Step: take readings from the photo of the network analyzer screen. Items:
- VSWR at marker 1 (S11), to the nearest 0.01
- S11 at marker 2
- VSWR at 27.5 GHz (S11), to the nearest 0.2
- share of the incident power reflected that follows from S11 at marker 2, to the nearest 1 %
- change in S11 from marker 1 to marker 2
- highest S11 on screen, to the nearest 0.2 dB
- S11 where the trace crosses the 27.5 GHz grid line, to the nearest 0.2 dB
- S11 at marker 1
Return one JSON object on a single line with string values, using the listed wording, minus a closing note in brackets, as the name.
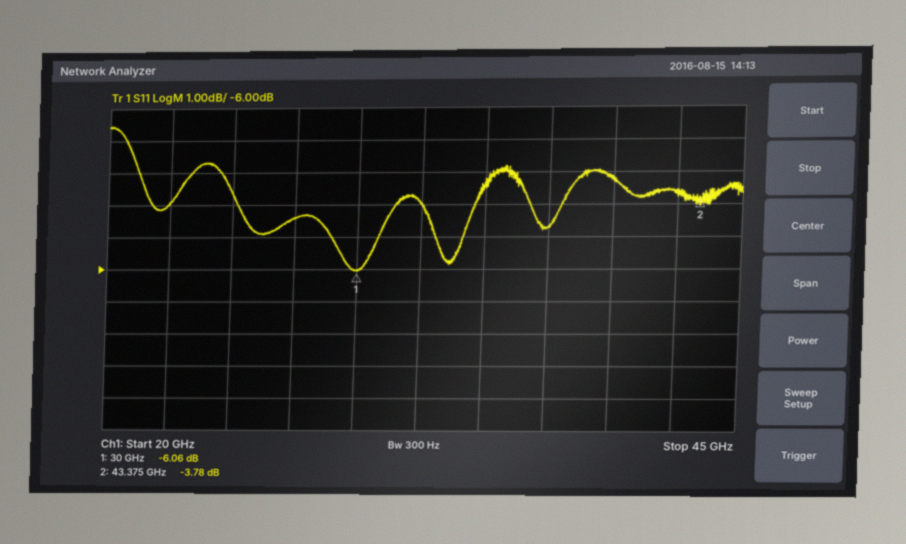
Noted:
{"VSWR at marker 1 (S11), to the nearest 0.01": "2.98", "S11 at marker 2": "-3.78 dB", "VSWR at 27.5 GHz (S11), to the nearest 0.2": "4.0", "share of the incident power reflected that follows from S11 at marker 2, to the nearest 1 %": "42 %", "change in S11 from marker 1 to marker 2": "2.28 dB", "highest S11 on screen, to the nearest 0.2 dB": "-1.6 dB", "S11 where the trace crosses the 27.5 GHz grid line, to the nearest 0.2 dB": "-4.4 dB", "S11 at marker 1": "-6.06 dB"}
